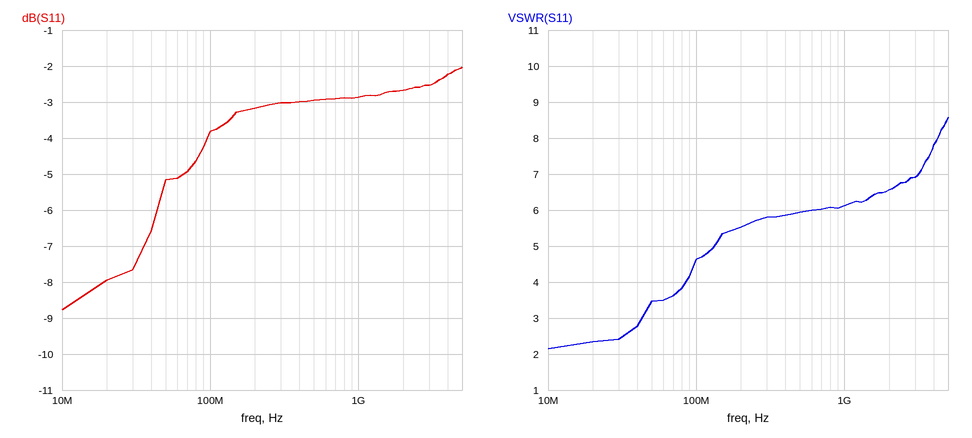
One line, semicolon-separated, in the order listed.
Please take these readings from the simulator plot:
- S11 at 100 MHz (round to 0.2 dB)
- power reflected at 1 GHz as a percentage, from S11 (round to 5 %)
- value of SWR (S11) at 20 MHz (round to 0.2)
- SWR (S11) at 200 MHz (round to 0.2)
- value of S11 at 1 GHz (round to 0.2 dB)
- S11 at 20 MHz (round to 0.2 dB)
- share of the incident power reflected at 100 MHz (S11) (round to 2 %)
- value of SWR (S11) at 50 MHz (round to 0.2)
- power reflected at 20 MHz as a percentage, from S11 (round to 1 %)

-3.8 dB; 50 %; 2.4; 5.6; -2.8 dB; -8.0 dB; 42 %; 3.4; 16 %
